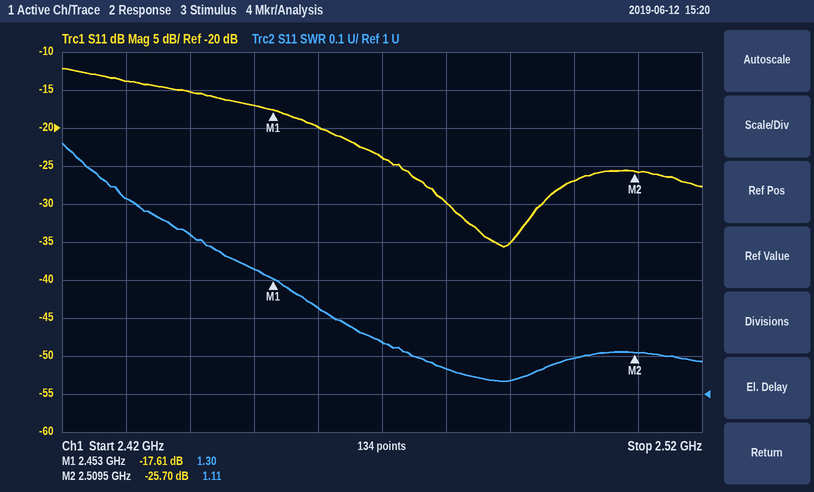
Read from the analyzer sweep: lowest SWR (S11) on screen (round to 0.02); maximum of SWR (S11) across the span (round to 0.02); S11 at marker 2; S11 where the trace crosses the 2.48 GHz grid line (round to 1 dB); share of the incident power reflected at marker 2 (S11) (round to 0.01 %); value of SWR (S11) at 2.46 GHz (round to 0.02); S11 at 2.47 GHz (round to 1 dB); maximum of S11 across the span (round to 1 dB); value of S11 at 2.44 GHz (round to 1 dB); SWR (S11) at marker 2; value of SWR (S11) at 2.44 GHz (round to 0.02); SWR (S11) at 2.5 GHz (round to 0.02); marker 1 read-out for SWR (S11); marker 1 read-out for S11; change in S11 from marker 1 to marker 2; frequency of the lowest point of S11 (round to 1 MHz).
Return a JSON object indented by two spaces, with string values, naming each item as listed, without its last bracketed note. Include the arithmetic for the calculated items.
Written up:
{
  "lowest SWR (S11) on screen": "1.04",
  "maximum of SWR (S11) across the span": "1.66",
  "S11 at marker 2": "-25.70 dB",
  "S11 where the trace crosses the 2.48 GHz grid line": "-30 dB",
  "share of the incident power reflected at marker 2 (S11)": "10^(-25.7/10) ≈ 0.27 %",
  "value of SWR (S11) at 2.46 GHz": "1.22",
  "S11 at 2.47 GHz": "-24 dB",
  "maximum of S11 across the span": "-12 dB",
  "value of S11 at 2.44 GHz": "-15 dB",
  "SWR (S11) at marker 2": "1.11",
  "value of SWR (S11) at 2.44 GHz": "1.42",
  "SWR (S11) at 2.5 GHz": "1.10",
  "marker 1 read-out for SWR": "1.30",
  "marker 1 read-out for S11": "-17.61 dB",
  "change in S11 from marker 1 to marker 2": "-25.7 − (-17.61) = -8.09 dB",
  "frequency of the lowest point of S11": "2.489 GHz"
}
